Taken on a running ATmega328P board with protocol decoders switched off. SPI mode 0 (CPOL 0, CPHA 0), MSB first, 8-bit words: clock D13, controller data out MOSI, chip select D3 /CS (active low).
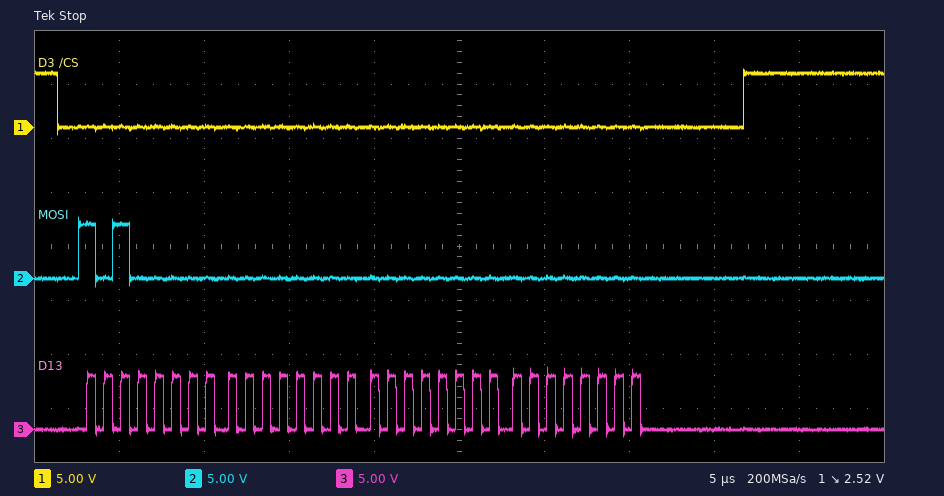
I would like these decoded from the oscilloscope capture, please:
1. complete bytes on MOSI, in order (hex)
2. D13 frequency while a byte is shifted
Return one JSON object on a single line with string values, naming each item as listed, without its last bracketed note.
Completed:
{"complete bytes on MOSI, in order": "A0 00 00 00", "D13 frequency while a byte is shifted": "1 MHz"}
